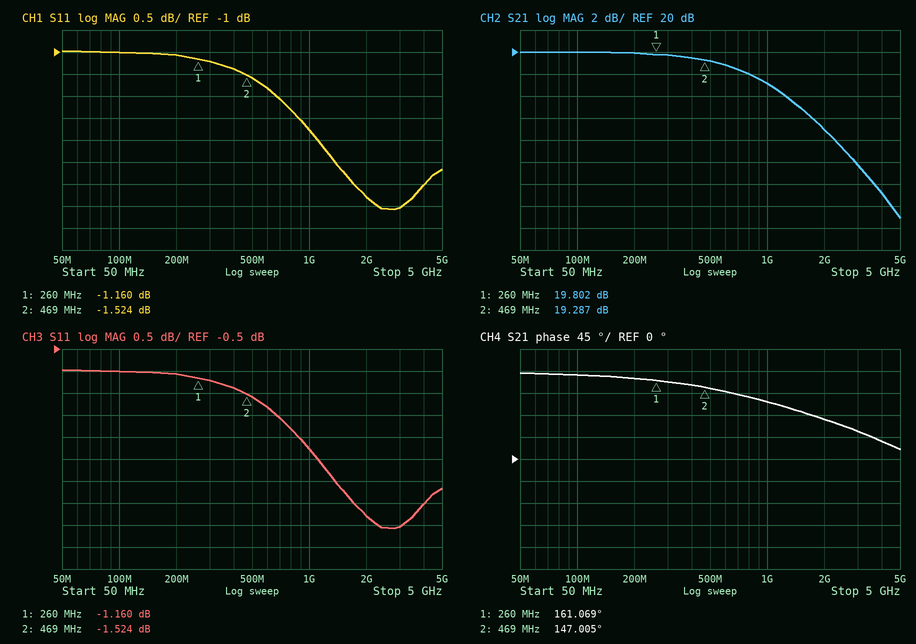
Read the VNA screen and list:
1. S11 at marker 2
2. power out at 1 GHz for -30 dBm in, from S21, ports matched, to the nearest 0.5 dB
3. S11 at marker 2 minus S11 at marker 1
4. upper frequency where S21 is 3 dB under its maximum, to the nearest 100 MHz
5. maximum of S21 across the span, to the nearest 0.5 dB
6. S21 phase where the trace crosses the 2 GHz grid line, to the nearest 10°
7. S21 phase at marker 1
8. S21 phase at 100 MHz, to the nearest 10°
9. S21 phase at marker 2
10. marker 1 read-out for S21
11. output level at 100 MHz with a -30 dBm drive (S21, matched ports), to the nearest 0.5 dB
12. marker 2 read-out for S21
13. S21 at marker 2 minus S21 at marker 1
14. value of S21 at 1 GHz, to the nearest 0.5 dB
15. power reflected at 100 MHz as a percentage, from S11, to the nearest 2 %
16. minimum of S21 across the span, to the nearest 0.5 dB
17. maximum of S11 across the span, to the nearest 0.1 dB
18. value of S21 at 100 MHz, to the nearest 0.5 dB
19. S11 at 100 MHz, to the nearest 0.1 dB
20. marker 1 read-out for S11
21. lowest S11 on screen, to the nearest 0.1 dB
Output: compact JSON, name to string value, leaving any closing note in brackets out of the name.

{"S11 at marker 2": "-1.524 dB", "power out at 1 GHz for -30 dBm in, from S21, ports matched, to the nearest 0.5 dB": "-13.0 dBm", "S11 at marker 2 minus S11 at marker 1": "-0.364 dB", "upper frequency where S21 is 3 dB under its maximum, to the nearest 100 MHz": "1.0 GHz", "maximum of S21 across the span, to the nearest 0.5 dB": "20.0 dB", "S21 phase where the trace crosses the 2 GHz grid line, to the nearest 10°": "80°", "S21 phase at marker 1": "161.069°", "S21 phase at 100 MHz, to the nearest 10°": "170°", "S21 phase at marker 2": "147.005°", "marker 1 read-out for S21": "19.802 dB", "output level at 100 MHz with a -30 dBm drive (S21, matched ports), to the nearest 0.5 dB": "-10.0 dBm", "marker 2 read-out for S21": "19.287 dB", "S21 at marker 2 minus S21 at marker 1": "-0.515 dB", "value of S21 at 1 GHz, to the nearest 0.5 dB": "17.0 dB", "power reflected at 100 MHz as a percentage, from S11, to the nearest 2 %": "80 %", "minimum of S21 across the span, to the nearest 0.5 dB": "5.0 dB", "maximum of S11 across the span, to the nearest 0.1 dB": "-1.0 dB", "value of S21 at 100 MHz, to the nearest 0.5 dB": "20.0 dB", "S11 at 100 MHz, to the nearest 0.1 dB": "-1.0 dB", "marker 1 read-out for S11": "-1.160 dB", "lowest S11 on screen, to the nearest 0.1 dB": "-4.6 dB"}
